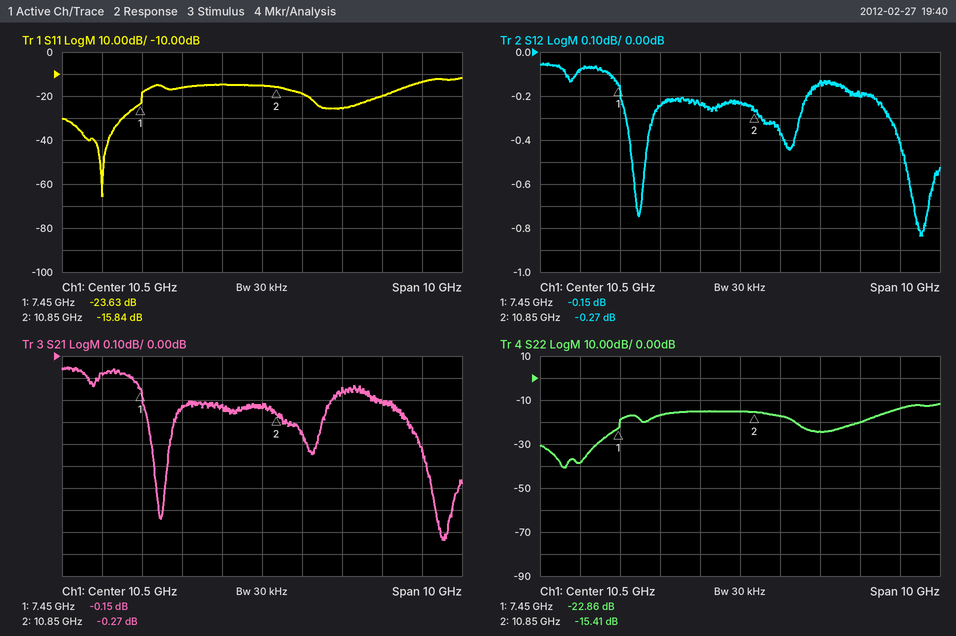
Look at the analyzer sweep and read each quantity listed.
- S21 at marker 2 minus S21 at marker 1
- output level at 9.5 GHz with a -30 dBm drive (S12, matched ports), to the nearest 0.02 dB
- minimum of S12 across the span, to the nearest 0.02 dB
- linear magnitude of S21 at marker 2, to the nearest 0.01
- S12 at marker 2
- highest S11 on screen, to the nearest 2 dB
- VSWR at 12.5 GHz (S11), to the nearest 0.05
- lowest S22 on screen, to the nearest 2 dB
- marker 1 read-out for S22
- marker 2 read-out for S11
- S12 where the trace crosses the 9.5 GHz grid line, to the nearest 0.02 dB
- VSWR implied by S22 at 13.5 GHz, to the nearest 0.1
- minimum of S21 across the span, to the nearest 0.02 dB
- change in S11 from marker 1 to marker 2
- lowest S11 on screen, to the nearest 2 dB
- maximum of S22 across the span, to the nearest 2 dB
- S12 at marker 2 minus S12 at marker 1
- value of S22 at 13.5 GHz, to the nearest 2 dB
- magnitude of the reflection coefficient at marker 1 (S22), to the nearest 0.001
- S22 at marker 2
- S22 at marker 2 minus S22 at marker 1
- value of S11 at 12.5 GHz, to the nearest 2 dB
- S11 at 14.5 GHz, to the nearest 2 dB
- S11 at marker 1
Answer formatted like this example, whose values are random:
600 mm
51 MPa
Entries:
-0.12 dB
-30.24 dBm
-0.84 dB
0.97
-0.27 dB
-12 dB
1.10
-40 dB
-22.86 dB
-15.84 dB
-0.24 dB
1.2
-0.84 dB
7.79 dB
-66 dB
-12 dB
-0.12 dB
-20 dB
0.072
-15.41 dB
7.45 dB
-26 dB
-14 dB
-23.63 dB
